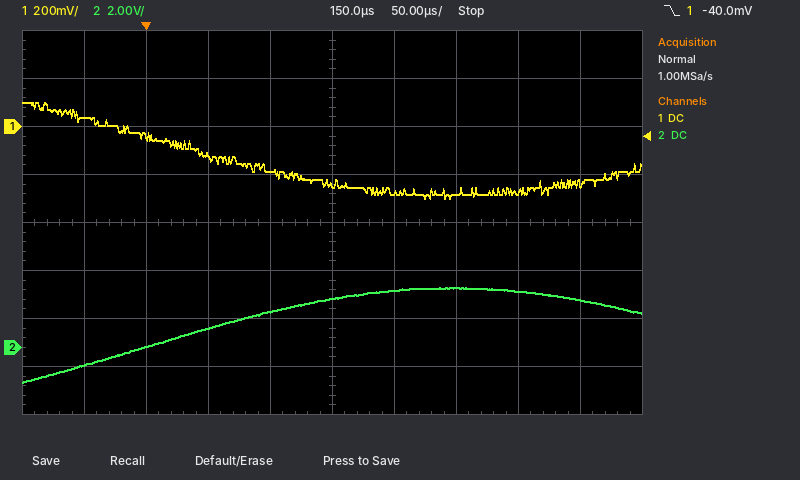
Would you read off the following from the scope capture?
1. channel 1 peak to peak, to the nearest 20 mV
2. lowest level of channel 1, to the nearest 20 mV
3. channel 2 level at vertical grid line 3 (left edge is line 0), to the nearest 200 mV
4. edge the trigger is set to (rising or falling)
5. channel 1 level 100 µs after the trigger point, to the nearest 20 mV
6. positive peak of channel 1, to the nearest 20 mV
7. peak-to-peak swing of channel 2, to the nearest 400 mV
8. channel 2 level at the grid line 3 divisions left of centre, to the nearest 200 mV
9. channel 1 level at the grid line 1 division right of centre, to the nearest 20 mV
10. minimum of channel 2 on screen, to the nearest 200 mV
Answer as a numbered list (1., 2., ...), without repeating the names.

1. 400 mV
2. -300 mV
3. 800 mV
4. falling
5. -180 mV
6. 100 mV
7. 4.0 V
8. 0.0 V
9. -280 mV
10. -1.4 V
